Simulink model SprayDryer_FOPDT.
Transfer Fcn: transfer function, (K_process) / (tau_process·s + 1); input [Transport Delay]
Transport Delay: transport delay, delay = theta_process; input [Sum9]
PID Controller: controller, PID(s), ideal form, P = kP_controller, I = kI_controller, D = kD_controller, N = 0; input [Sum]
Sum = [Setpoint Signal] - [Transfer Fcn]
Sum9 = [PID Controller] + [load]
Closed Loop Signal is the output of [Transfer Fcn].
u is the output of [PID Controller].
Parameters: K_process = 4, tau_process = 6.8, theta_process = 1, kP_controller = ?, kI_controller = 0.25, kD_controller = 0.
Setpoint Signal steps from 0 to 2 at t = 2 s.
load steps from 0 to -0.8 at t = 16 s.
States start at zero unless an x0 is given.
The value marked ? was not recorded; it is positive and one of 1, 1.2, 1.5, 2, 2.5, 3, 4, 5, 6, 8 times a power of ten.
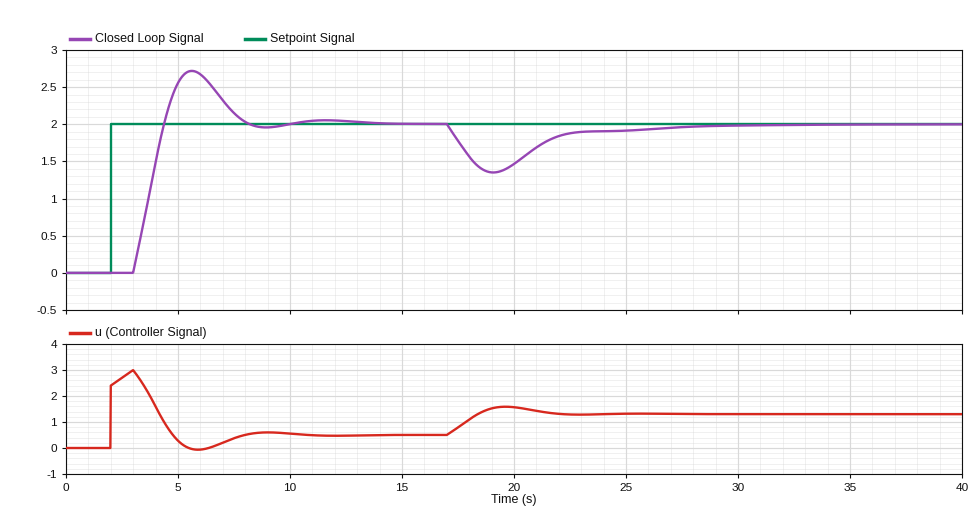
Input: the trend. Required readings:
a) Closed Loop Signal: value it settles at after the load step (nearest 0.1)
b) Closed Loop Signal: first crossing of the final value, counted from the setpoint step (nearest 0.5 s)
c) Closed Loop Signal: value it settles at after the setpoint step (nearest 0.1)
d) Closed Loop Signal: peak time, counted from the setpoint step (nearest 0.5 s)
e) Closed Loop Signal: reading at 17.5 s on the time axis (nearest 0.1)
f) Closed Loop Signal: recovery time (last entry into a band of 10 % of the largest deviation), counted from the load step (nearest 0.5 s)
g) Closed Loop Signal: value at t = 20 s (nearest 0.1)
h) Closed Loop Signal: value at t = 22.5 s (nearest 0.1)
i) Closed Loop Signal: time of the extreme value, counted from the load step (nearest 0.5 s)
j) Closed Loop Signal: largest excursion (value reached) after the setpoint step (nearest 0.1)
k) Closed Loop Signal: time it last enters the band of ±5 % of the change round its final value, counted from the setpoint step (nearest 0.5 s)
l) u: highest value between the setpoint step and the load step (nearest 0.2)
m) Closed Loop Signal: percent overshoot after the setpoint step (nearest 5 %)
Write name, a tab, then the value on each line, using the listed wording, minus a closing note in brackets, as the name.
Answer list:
Closed Loop Signal: value it settles at after the load step	2.0
Closed Loop Signal: first crossing of the final value, counted from the setpoint step	2.5 s
Closed Loop Signal: value it settles at after the setpoint step	2.0
Closed Loop Signal: peak time, counted from the setpoint step	3.5 s
Closed Loop Signal: reading at 17.5 s on the time axis	1.8
Closed Loop Signal: recovery time (last entry into a band of 10 % of the largest deviation), counted from the load step	10.0 s
Closed Loop Signal: value at t = 20 s	1.5
Closed Loop Signal: value at t = 22.5 s	1.9
Closed Loop Signal: time of the extreme value, counted from the load step	3.0 s
Closed Loop Signal: largest excursion (value reached) after the setpoint step	2.7
Closed Loop Signal: time it last enters the band of ±5 % of the change round its final value, counted from the setpoint step	5.5 s
u: highest value between the setpoint step and the load step	3.0
Closed Loop Signal: percent overshoot after the setpoint step	35 %
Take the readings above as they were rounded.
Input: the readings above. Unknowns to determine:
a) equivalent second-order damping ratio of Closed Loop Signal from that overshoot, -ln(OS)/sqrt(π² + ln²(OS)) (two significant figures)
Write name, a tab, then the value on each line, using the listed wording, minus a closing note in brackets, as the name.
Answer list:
equivalent second-order damping ratio of Closed Loop Signal from that overshoot, -ln(OS)/sqrt(π² + ln²(OS))	0.32
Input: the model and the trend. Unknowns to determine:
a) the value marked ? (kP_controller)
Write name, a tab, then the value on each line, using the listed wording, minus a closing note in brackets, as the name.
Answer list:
the value marked ?	1.2
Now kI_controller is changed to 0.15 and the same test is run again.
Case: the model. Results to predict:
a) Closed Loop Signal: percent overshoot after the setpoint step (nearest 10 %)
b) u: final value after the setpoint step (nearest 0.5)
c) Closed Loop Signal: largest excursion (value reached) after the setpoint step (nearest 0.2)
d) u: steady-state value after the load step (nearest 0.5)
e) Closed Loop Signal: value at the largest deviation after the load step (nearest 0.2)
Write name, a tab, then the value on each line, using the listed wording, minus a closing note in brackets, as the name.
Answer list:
Closed Loop Signal: percent overshoot after the setpoint step	20 %
u: final value after the setpoint step	0.5
Closed Loop Signal: largest excursion (value reached) after the setpoint step	2.4
u: steady-state value after the load step	1.5
Closed Loop Signal: value at the largest deviation after the load step	1.4
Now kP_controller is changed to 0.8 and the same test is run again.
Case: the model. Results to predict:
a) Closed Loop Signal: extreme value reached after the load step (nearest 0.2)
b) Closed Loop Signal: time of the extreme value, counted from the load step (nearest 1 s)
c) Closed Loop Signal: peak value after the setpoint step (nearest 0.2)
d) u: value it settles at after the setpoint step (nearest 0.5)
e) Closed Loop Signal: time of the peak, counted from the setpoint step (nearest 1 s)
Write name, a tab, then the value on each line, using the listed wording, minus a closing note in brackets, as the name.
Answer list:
Closed Loop Signal: extreme value reached after the load step	1.2
Closed Loop Signal: time of the extreme value, counted from the load step	4 s
Closed Loop Signal: peak value after the setpoint step	2.4
u: value it settles at after the setpoint step	0.5
Closed Loop Signal: time of the peak, counted from the setpoint step	5 s
